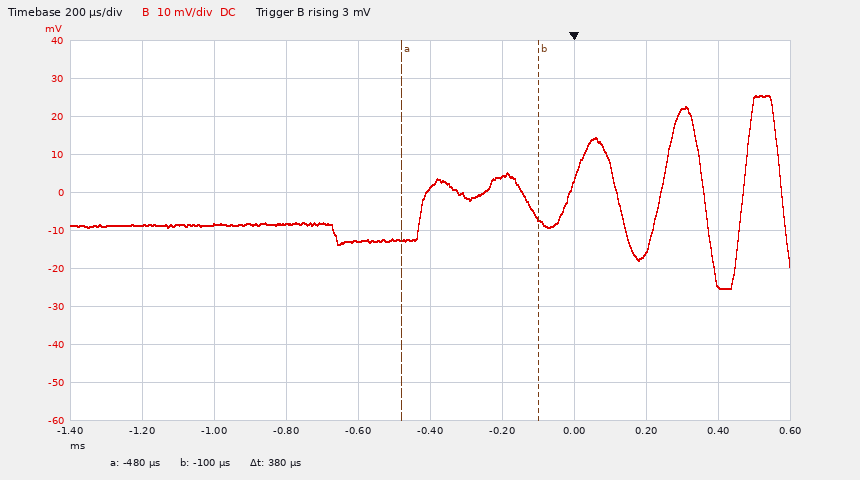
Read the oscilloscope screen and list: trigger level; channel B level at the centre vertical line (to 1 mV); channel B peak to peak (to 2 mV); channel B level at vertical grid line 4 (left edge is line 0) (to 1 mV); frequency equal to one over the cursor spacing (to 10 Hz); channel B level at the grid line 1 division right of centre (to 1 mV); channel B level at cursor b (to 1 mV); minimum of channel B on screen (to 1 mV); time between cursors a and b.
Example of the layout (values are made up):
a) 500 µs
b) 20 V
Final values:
a) 3 mV
b) 1 mV
c) 50 mV
d) -13 mV
e) 2.63 kHz
f) 4 mV
g) -7 mV
h) -25 mV
i) 380 µs
